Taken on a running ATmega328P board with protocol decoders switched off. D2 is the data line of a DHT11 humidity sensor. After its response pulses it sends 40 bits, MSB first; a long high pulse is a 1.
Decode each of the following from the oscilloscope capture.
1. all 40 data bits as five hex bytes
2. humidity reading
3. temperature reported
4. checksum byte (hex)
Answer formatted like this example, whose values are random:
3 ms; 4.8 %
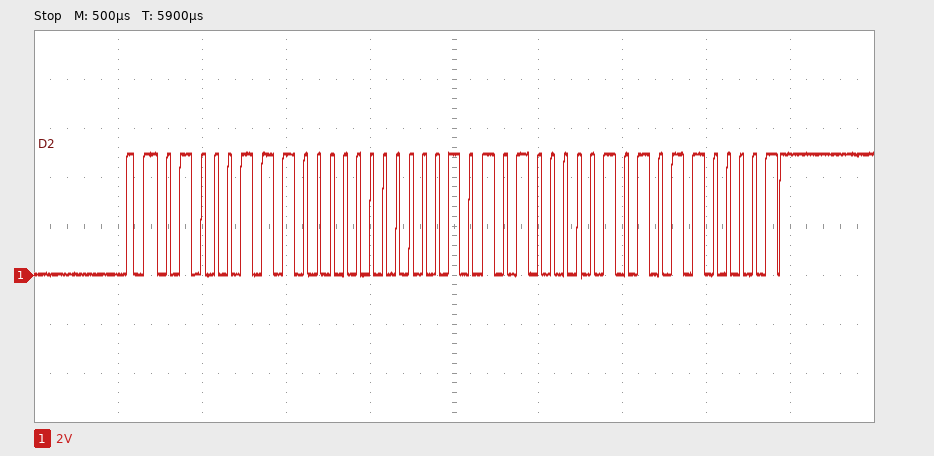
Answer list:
47 00 15 05 61; 71 %; 21.5 °C; 0x61
